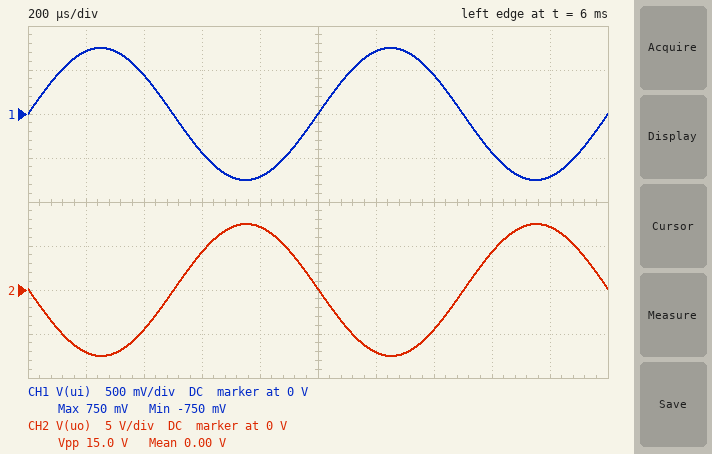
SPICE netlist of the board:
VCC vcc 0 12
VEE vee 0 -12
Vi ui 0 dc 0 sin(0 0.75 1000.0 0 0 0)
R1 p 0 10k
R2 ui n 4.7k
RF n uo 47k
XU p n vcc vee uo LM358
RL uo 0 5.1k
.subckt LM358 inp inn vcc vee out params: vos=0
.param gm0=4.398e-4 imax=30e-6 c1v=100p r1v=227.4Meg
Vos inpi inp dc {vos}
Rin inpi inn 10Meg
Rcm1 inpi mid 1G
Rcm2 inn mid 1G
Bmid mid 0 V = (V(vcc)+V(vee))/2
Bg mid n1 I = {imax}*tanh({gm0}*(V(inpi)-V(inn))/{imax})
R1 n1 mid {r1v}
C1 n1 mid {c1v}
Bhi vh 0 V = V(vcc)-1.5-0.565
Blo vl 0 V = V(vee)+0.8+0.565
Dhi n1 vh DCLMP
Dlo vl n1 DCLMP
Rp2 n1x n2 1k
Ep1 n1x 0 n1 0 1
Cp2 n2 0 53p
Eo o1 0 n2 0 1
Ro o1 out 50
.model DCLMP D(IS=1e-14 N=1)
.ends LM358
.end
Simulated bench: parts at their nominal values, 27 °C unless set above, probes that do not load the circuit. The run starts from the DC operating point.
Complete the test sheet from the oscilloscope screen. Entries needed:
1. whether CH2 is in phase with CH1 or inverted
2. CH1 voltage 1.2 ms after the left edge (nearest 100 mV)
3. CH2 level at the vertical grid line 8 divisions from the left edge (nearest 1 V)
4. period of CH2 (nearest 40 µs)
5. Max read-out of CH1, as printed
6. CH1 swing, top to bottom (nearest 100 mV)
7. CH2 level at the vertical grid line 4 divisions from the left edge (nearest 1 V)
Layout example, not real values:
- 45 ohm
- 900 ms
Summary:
- inverted
- 700 mV
- 4 V
- 1.00 ms
- 750 mV
- 1.5 V
- 7 V
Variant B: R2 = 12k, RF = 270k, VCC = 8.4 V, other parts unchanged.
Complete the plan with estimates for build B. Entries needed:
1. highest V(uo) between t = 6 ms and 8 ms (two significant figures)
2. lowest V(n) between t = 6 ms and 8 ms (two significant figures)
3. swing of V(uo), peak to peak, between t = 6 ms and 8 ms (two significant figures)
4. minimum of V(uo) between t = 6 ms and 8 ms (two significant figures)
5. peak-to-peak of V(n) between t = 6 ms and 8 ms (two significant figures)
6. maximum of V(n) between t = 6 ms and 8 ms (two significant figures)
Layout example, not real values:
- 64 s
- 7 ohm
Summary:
- 6.8 V
- -430 mV
- 18 V
- -11 V
- 670 mV
- 250 mV
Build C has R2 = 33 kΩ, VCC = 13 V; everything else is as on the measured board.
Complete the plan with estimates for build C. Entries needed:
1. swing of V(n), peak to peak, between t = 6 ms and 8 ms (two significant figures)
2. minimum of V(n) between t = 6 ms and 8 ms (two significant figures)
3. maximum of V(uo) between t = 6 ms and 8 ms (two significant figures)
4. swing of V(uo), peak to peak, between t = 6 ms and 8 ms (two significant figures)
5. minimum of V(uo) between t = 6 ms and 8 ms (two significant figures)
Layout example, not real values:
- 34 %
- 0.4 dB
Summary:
- 3.1 mV
- -1.5 mV
- 1.1 V
- 2.1 V
- -1.1 V
